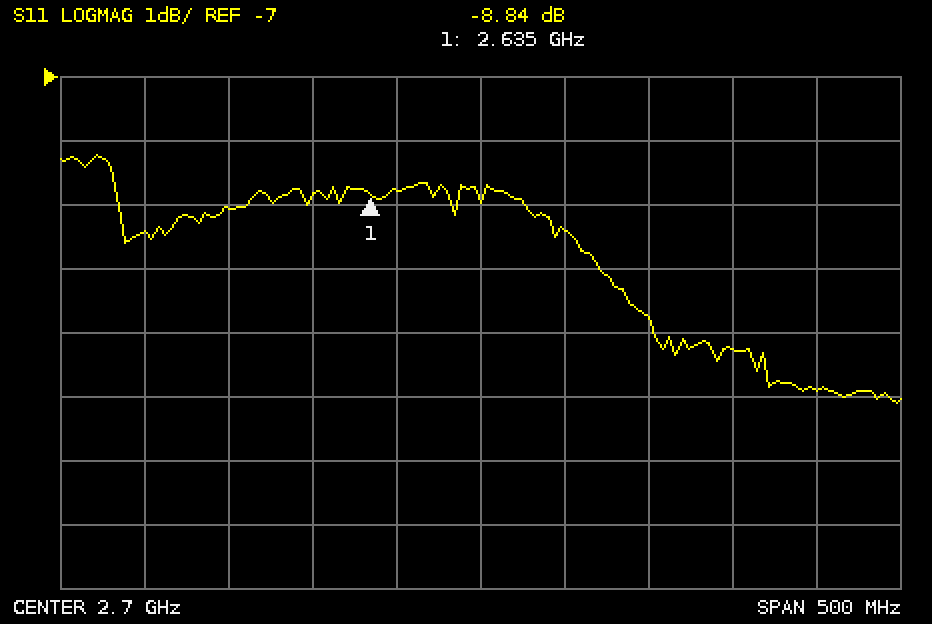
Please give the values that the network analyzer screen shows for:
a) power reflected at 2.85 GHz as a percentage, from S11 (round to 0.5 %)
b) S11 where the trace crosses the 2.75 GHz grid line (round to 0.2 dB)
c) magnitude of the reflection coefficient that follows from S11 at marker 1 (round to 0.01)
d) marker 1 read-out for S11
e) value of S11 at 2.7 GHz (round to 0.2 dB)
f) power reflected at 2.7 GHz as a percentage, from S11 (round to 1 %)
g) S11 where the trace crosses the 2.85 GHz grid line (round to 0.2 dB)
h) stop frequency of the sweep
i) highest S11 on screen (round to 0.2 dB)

7.5 %
-9.4 dB
0.36
-8.84 dB
-9.0 dB
13 %
-11.2 dB
2.95 GHz
-8.2 dB
